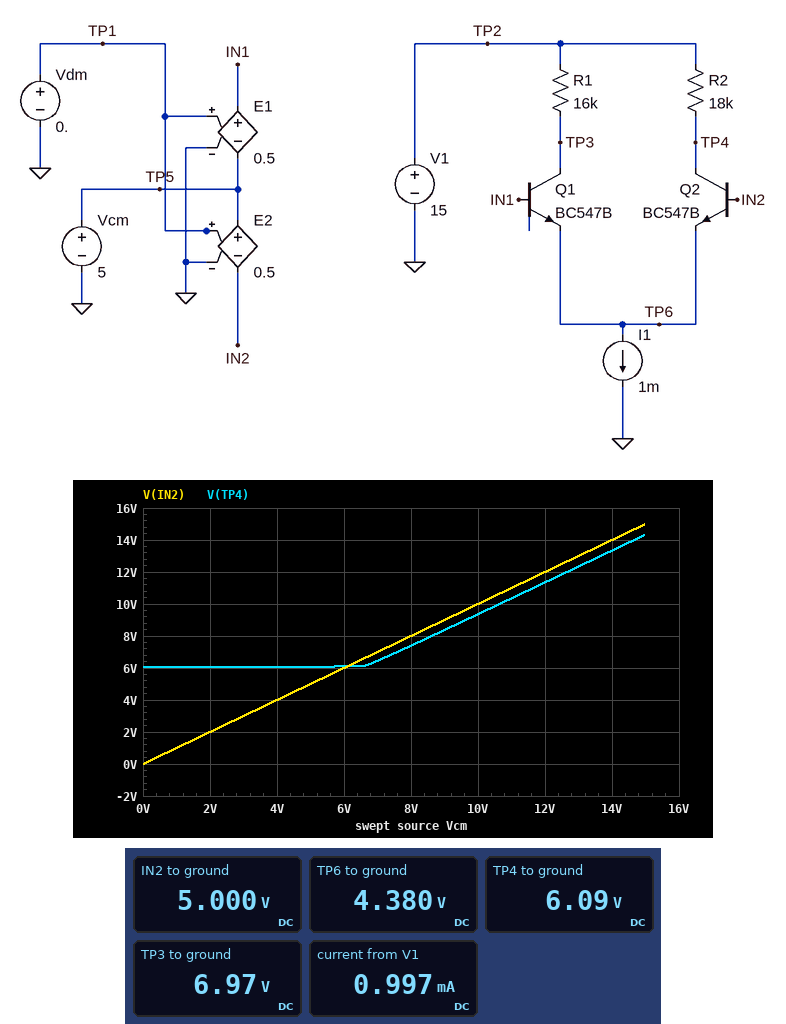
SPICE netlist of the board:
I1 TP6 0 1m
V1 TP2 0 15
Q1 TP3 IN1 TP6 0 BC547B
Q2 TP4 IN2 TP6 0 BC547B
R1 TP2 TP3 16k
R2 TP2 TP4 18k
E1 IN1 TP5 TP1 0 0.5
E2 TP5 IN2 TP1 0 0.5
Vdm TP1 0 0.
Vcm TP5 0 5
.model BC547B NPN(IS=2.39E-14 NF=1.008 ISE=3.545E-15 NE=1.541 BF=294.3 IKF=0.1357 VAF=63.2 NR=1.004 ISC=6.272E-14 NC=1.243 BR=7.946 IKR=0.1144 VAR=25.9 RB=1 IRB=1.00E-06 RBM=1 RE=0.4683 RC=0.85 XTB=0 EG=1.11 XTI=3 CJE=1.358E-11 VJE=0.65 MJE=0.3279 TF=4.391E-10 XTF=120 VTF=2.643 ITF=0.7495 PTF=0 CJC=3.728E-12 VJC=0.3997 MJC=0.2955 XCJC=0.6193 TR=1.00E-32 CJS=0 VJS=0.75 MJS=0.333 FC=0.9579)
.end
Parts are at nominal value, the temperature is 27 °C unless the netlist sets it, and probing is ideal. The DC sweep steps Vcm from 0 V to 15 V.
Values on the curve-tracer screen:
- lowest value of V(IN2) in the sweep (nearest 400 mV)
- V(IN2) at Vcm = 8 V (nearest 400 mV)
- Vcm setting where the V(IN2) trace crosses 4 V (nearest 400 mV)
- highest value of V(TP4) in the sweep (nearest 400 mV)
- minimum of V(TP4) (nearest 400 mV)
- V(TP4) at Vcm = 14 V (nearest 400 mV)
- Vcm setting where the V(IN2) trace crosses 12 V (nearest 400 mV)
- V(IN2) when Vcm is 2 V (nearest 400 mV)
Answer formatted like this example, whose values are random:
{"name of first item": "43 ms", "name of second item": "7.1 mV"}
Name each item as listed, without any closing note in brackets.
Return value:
{"lowest value of V(IN2) in the sweep": "0 V", "V(IN2) at Vcm = 8 V": "8.0 V", "Vcm setting where the V(IN2) trace crosses 4 V": "4.0 V", "highest value of V(TP4) in the sweep": "14.4 V", "minimum of V(TP4)": "6.0 V", "V(TP4) at Vcm = 14 V": "13.2 V", "Vcm setting where the V(IN2) trace crosses 12 V": "12.0 V", "V(IN2) when Vcm is 2 V": "2.0 V"}
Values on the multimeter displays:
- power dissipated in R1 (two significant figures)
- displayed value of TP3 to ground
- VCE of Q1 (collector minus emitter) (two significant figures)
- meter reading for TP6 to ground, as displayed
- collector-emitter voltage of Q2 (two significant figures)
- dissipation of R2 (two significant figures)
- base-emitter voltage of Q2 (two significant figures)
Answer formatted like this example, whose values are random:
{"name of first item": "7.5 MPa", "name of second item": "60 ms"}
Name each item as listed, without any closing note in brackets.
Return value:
{"power dissipated in R1": "4.0 mW", "displayed value of TP3 to ground": "6.97 V", "VCE of Q1 (collector minus emitter)": "2.6 V", "meter reading for TP6 to ground, as displayed": "4.380 V", "collector-emitter voltage of Q2": "1.7 V", "dissipation of R2": "4.4 mW", "base-emitter voltage of Q2": "620 mV"}
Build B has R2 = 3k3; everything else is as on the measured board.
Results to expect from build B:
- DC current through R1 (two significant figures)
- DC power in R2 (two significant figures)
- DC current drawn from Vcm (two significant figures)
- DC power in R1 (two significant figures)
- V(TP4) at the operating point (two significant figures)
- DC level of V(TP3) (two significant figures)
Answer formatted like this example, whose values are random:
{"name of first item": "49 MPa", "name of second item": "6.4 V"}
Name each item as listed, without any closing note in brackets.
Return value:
{"DC current through R1": "480 µA", "DC power in R2": "890 µW", "DC current drawn from Vcm": "3.2 µA", "DC power in R1": "3.6 mW", "V(TP4) at the operating point": "13 V", "DC level of V(TP3)": "7.4 V"}
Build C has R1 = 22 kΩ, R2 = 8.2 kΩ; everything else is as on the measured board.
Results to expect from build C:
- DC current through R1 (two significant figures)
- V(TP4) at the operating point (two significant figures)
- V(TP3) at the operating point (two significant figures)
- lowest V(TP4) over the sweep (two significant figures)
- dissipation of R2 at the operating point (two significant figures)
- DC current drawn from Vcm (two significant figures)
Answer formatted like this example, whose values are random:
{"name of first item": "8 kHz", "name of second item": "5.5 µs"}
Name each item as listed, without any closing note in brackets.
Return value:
{"DC current through R1": "470 µA", "V(TP4) at the operating point": "11 V", "V(TP3) at the operating point": "4.6 V", "lowest V(TP4) over the sweep": "9.4 V", "dissipation of R2 at the operating point": "2.2 mW", "DC current drawn from Vcm": "3.5 µA"}
